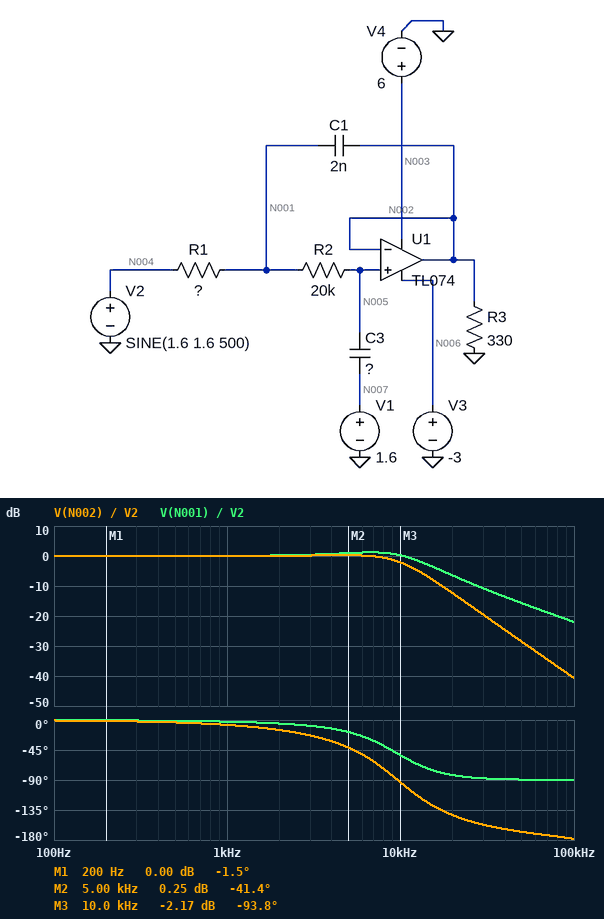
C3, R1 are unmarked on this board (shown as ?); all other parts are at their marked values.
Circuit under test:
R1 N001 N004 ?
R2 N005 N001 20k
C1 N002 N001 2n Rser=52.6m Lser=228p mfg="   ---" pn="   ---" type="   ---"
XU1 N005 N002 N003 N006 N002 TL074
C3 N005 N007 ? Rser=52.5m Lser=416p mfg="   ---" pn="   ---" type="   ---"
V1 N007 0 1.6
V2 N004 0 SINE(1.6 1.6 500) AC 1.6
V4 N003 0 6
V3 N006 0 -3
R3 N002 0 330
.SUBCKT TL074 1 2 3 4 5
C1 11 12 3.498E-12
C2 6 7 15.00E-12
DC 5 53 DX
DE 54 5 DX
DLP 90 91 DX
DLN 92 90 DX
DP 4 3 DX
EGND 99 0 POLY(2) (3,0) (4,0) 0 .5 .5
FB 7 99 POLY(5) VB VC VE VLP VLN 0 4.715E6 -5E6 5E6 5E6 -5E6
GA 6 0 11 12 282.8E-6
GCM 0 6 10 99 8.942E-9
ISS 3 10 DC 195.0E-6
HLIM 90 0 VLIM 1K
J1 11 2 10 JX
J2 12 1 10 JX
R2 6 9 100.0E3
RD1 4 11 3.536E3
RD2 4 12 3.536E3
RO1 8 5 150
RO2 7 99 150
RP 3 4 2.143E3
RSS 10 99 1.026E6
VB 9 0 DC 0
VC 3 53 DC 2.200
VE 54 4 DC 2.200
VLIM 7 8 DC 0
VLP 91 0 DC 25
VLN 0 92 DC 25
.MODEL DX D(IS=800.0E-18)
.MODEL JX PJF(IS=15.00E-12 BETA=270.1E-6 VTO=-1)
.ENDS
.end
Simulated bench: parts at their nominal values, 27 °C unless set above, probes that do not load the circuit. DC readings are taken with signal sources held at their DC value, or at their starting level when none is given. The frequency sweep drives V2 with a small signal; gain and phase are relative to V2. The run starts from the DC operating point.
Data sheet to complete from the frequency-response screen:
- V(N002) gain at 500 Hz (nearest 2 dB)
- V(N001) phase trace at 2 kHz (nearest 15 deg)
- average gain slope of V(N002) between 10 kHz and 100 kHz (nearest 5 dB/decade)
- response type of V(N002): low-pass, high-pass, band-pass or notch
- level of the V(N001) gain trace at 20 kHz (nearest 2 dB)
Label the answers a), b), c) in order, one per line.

a) 0 dB
b) 0 deg
c) -40 dB/decade
d) low-pass
e) -6 dB
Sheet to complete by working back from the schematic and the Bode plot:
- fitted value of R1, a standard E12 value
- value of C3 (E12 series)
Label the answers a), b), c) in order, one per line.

a) 10 kΩ
b) 680 pF
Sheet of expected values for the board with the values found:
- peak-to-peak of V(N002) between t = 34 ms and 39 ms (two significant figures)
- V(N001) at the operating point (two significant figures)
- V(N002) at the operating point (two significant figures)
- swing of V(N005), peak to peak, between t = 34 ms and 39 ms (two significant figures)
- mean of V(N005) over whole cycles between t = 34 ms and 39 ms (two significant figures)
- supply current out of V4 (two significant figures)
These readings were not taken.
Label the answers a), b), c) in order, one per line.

a) 3.2 V
b) 1.6 V
c) 1.6 V
d) 3.2 V
e) 1.6 V
f) 4.4 mA
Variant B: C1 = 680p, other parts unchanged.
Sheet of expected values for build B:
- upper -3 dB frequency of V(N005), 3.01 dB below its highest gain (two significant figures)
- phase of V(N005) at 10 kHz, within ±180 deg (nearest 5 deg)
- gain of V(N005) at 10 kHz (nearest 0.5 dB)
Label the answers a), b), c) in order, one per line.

a) 9.8 kHz
b) -65 deg
c) -3.0 dB
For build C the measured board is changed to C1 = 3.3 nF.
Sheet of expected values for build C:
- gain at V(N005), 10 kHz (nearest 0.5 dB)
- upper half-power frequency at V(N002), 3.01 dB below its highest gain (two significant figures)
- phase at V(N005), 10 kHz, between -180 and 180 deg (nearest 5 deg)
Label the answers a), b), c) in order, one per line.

a) -3.5 dB
b) 8.8 kHz
c) -120 deg
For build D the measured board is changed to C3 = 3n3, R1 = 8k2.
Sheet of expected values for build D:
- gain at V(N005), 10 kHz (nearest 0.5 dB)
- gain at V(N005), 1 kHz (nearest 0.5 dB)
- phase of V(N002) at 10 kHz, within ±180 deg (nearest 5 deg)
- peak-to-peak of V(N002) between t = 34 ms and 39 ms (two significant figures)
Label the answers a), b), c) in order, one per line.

a) -16.5 dB
b) -1.0 dB
c) -120 deg
d) 3.1 V
